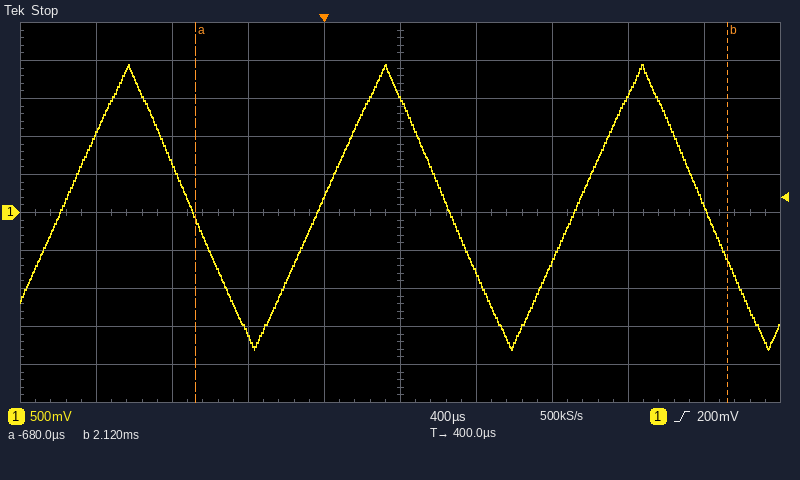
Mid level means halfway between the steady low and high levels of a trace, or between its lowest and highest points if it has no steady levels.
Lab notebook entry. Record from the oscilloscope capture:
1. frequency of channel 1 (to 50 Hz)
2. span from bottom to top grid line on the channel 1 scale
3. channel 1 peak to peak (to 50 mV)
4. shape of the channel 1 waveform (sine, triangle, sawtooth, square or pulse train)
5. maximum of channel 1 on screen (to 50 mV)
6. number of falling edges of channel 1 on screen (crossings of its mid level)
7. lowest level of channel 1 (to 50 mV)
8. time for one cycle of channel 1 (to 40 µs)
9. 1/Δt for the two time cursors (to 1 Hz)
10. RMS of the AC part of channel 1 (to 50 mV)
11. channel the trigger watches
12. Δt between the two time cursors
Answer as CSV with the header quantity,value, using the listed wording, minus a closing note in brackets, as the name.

quantity,value
frequency of channel 1,750 Hz
span from bottom to top grid line on the channel 1 scale,5 V
channel 1 peak to peak,3.75 V
shape of the channel 1 waveform,triangle
maximum of channel 1 on screen,1.95 V
number of falling edges of channel 1 on screen,3
lowest level of channel 1,-1.80 V
time for one cycle of channel 1,1.36 ms
1/Δt for the two time cursors,357 Hz
RMS of the AC part of channel 1,1.10 V
channel the trigger watches,channel 1
Δt between the two time cursors,2.80 ms
